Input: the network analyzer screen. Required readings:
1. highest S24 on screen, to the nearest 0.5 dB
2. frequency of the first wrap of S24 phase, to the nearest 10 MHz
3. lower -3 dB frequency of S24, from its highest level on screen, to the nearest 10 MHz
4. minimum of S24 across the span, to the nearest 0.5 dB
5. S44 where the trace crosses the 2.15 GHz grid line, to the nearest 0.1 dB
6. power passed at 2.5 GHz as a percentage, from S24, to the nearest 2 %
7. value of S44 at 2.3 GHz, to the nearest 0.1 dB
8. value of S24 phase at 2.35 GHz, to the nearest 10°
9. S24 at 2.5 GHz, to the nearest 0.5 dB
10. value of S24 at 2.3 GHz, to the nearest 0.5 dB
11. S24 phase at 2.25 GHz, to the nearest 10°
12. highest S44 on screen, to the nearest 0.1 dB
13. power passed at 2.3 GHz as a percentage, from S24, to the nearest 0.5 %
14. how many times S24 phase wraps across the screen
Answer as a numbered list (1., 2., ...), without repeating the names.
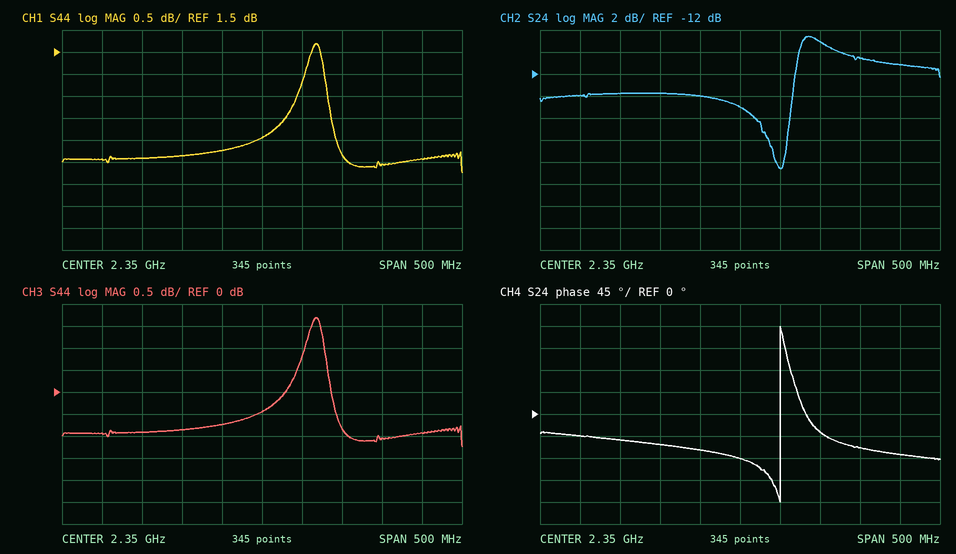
1. -8.5 dB
2. 2.40 GHz
3. 2.42 GHz
4. -20.5 dB
5. -0.9 dB
6. 8 %
7. -0.7 dB
8. -90°
9. -10.5 dB
10. -14.0 dB
11. -60°
12. 1.7 dB
13. 4.0 %
14. 1
